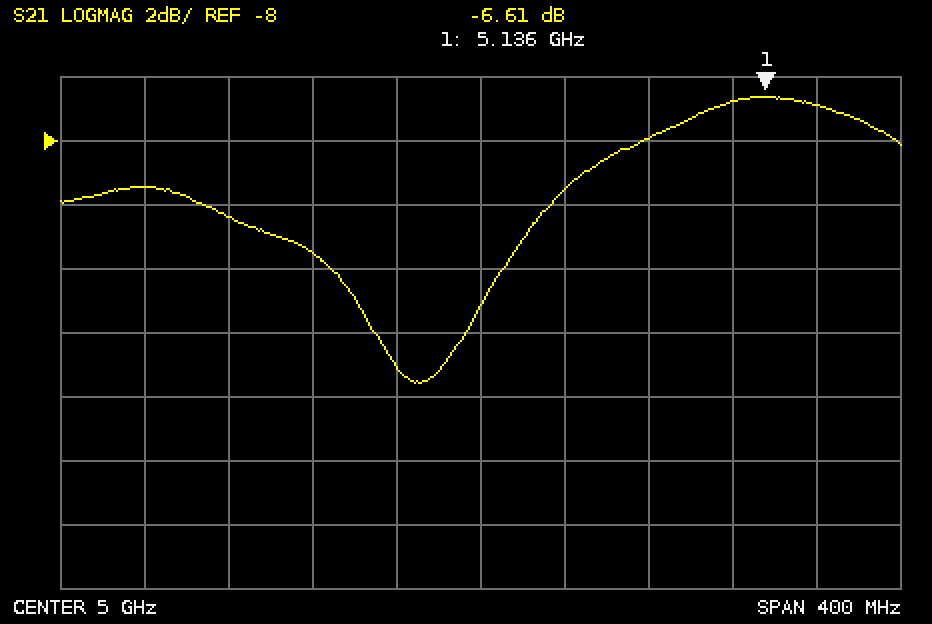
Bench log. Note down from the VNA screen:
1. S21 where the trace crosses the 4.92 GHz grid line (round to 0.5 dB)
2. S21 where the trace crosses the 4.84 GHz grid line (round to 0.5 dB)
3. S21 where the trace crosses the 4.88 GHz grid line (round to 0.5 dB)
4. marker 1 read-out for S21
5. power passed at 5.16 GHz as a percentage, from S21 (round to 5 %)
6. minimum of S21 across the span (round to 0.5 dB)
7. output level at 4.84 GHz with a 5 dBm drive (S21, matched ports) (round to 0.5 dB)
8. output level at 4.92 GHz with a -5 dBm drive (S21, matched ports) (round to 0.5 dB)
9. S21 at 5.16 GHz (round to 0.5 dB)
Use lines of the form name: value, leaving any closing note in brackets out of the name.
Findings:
S21 where the trace crosses the 4.92 GHz grid line: -11.5 dB
S21 where the trace crosses the 4.84 GHz grid line: -9.5 dB
S21 where the trace crosses the 4.88 GHz grid line: -10.5 dB
marker 1 read-out for S21: -6.61 dB
power passed at 5.16 GHz as a percentage, from S21: 20 %
minimum of S21 across the span: -15.5 dB
output level at 4.84 GHz with a 5 dBm drive (S21, matched ports): -4.5 dBm
output level at 4.92 GHz with a -5 dBm drive (S21, matched ports): -16.5 dBm
S21 at 5.16 GHz: -7.0 dB
